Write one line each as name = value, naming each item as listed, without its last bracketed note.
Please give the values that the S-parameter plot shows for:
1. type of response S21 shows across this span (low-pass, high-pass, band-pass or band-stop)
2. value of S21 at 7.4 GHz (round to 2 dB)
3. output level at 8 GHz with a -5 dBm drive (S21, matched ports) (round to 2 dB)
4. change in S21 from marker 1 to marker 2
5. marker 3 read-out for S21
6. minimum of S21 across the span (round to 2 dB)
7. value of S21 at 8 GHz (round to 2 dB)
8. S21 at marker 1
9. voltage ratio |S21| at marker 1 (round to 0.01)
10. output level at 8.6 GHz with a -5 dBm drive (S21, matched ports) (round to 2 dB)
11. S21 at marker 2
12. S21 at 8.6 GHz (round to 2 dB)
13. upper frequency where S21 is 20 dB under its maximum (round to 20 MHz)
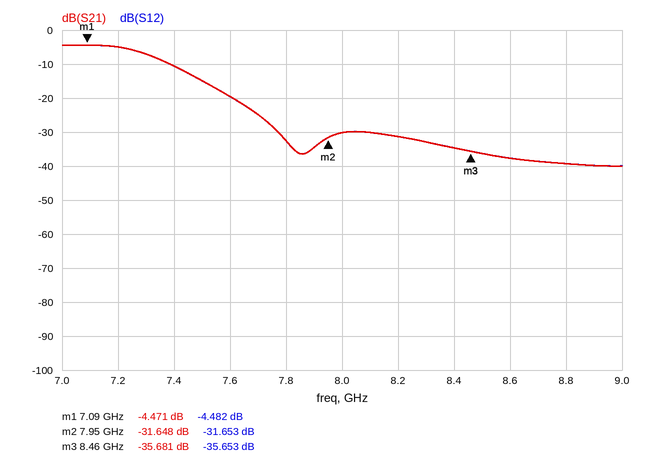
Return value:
type of response S21 shows across this span = low-pass
value of S21 at 7.4 GHz = -10 dB
output level at 8 GHz with a -5 dBm drive (S21, matched ports) = -36 dBm
change in S21 from marker 1 to marker 2 = -27.177 dB
marker 3 read-out for S21 = -35.681 dB
minimum of S21 across the span = -40 dB
value of S21 at 8 GHz = -30 dB
S21 at marker 1 = -4.471 dB
voltage ratio |S21| at marker 1 = 0.60
output level at 8.6 GHz with a -5 dBm drive (S21, matched ports) = -42 dBm
S21 at marker 2 = -31.648 dB
S21 at 8.6 GHz = -38 dB
upper frequency where S21 is 20 dB under its maximum = 7.70 GHz
